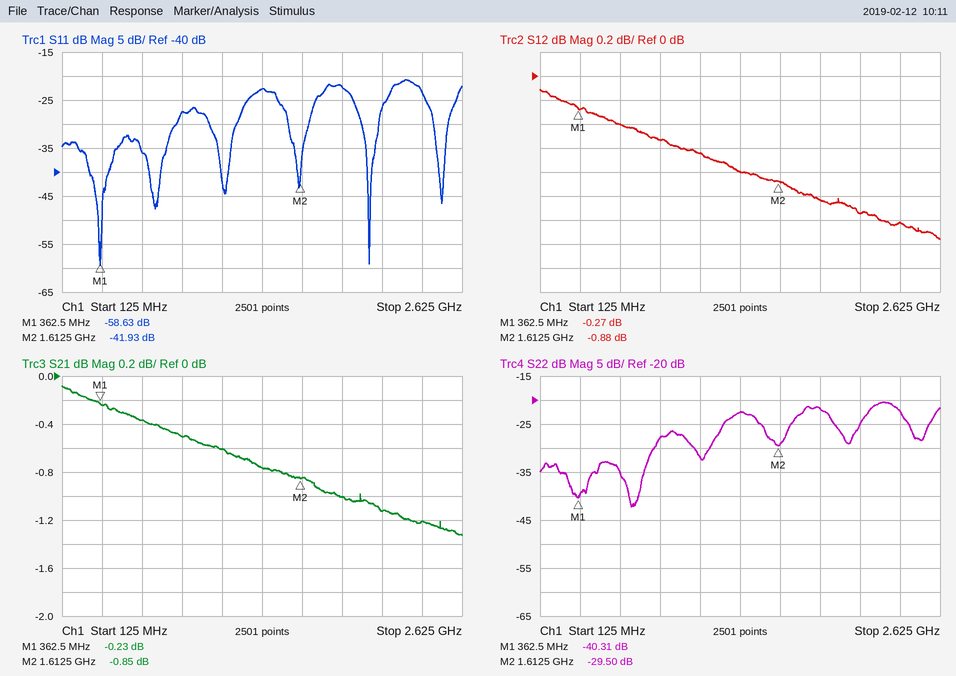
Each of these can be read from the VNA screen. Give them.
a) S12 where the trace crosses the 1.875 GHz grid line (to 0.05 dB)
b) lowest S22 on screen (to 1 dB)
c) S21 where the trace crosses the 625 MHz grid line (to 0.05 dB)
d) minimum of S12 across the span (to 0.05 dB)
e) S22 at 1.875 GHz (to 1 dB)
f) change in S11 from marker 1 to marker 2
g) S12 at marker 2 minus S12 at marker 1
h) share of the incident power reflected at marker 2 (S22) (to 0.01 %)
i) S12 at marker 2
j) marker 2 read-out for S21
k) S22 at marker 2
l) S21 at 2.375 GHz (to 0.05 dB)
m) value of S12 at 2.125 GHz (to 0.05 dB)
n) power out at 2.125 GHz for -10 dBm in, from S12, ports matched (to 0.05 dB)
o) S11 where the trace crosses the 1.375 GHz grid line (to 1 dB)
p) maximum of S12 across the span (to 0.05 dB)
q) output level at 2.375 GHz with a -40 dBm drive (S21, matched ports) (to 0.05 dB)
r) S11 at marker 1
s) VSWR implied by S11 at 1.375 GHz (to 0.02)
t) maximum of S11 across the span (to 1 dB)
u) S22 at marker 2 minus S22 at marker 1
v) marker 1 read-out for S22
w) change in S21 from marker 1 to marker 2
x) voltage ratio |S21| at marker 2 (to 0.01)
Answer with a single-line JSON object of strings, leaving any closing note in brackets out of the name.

{"S12 where the trace crosses the 1.875 GHz grid line": "-1.05 dB", "lowest S22 on screen": "-42 dB", "S21 where the trace crosses the 625 MHz grid line": "-0.35 dB", "minimum of S12 across the span": "-1.35 dB", "S22 at 1.875 GHz": "-22 dB", "change in S11 from marker 1 to marker 2": "16.70 dB", "S12 at marker 2 minus S12 at marker 1": "-0.61 dB", "share of the incident power reflected at marker 2 (S22)": "0.11 %", "S12 at marker 2": "-0.88 dB", "marker 2 read-out for S21": "-0.85 dB", "S22 at marker 2": "-29.50 dB", "S21 at 2.375 GHz": "-1.20 dB", "value of S12 at 2.125 GHz": "-1.15 dB", "power out at 2.125 GHz for -10 dBm in, from S12, ports matched": "-11.15 dBm", "S11 where the trace crosses the 1.375 GHz grid line": "-23 dB", "maximum of S12 across the span": "-0.10 dB", "output level at 2.375 GHz with a -40 dBm drive (S21, matched ports)": "-41.20 dBm", "S11 at marker 1": "-58.63 dB", "VSWR implied by S11 at 1.375 GHz": "1.16", "maximum of S11 across the span": "-21 dB", "S22 at marker 2 minus S22 at marker 1": "10.81 dB", "marker 1 read-out for S22": "-40.31 dB", "change in S21 from marker 1 to marker 2": "-0.62 dB", "voltage ratio |S21| at marker 2": "0.91"}
